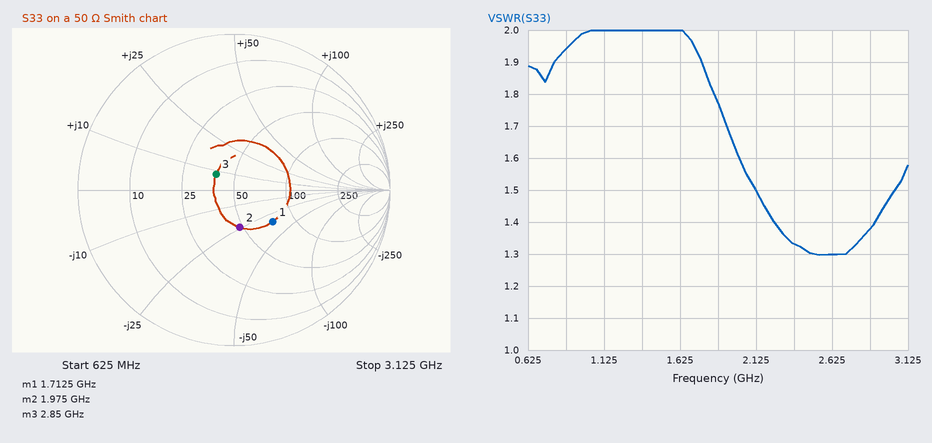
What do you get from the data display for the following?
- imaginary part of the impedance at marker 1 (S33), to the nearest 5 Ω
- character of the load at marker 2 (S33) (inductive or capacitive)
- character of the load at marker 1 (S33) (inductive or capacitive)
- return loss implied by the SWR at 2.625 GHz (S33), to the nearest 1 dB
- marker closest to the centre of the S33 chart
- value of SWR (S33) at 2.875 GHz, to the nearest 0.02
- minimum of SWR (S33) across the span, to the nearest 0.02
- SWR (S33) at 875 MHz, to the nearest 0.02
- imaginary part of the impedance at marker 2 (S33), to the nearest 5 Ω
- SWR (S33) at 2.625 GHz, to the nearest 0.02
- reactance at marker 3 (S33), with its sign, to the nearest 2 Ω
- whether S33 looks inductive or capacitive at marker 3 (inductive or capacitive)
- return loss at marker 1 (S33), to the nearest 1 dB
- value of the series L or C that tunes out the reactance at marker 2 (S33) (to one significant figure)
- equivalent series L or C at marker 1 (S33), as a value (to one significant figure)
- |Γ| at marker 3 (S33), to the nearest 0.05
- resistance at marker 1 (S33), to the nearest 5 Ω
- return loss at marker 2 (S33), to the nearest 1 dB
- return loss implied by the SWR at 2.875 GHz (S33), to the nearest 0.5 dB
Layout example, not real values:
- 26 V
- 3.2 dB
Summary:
- -35 Ω
- capacitive
- capacitive
- 18 dB
- marker 3
- 1.38
- 1.30
- 1.94
- -25 Ω
- 1.30
- +8 Ω
- inductive
- 10 dB
- 2 nH
- 3 pF
- 0.15
- 75 Ω
- 12 dB
- 16.0 dB
